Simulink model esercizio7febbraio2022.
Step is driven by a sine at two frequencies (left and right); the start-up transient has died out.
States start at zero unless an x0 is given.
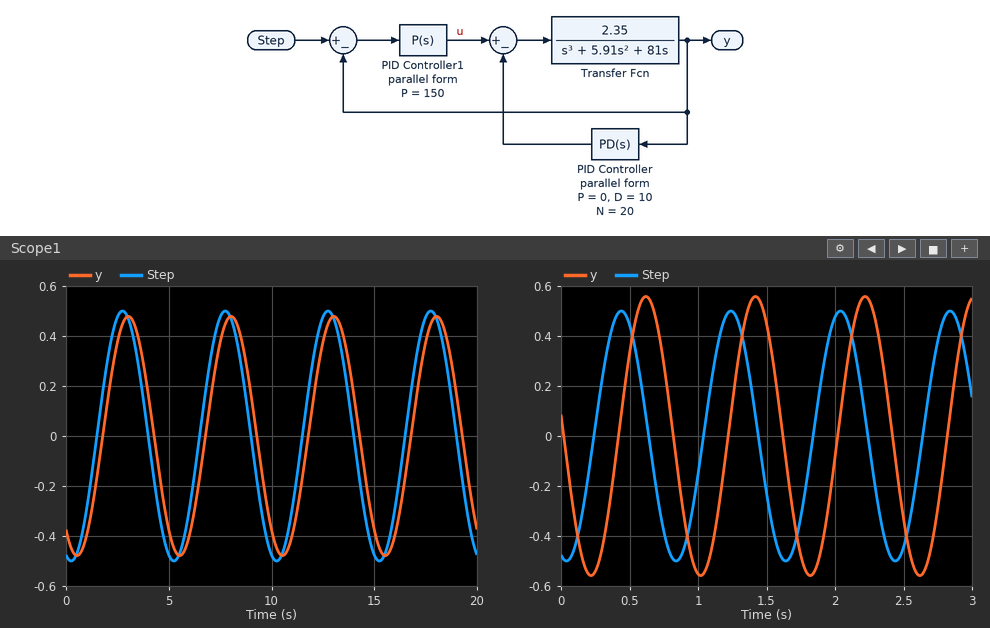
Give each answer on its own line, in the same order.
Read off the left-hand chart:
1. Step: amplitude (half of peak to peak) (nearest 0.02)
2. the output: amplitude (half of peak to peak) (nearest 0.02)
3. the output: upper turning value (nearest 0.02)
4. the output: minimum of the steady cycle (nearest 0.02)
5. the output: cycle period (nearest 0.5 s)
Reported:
0.50
0.48
0.48
-0.48
5.0 s
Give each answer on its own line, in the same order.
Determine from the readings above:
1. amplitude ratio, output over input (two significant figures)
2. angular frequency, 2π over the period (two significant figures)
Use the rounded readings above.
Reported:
0.96
1.3 rad/s
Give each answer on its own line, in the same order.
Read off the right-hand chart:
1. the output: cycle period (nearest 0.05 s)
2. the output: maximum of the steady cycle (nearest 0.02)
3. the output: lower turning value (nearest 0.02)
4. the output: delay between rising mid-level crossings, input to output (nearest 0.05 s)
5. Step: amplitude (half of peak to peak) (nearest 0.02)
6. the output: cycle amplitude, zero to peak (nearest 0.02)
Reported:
0.80 s
0.56
-0.56
0.20 s
0.50
0.56
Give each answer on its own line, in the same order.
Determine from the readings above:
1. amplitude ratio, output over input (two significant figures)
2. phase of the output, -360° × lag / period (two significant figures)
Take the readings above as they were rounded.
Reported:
1.1
-90°
